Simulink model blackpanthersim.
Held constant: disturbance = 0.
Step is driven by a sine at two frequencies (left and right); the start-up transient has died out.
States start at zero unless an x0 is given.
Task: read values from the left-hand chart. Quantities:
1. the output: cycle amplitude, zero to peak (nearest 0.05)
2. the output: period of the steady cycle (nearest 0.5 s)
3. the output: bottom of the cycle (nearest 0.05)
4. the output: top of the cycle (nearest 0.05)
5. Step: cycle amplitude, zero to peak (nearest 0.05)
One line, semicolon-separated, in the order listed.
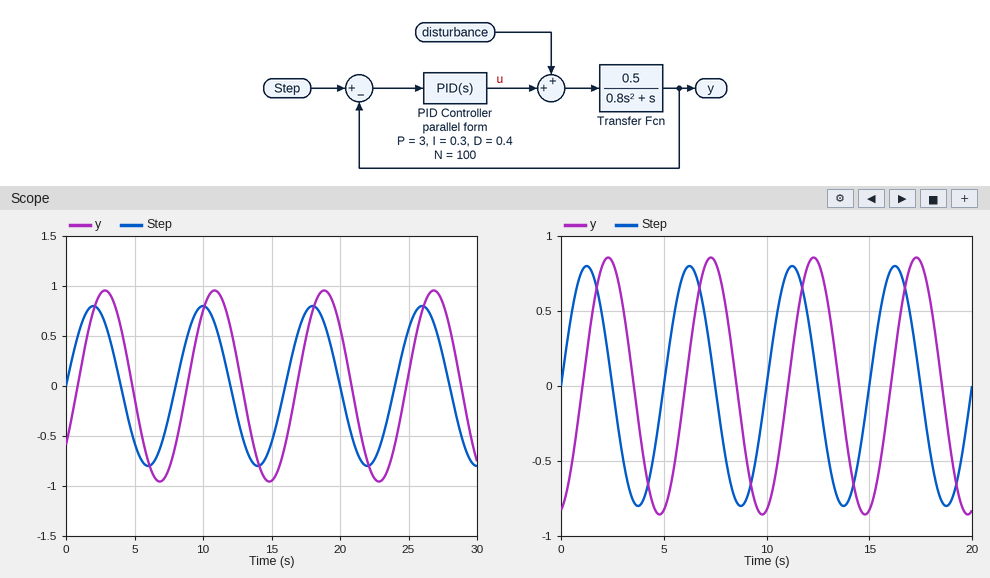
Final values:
0.95; 8.0 s; -0.95; 0.95; 0.80
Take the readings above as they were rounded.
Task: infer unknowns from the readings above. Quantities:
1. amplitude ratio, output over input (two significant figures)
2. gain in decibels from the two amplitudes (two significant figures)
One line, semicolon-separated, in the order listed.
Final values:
1.2; 1.5 dB
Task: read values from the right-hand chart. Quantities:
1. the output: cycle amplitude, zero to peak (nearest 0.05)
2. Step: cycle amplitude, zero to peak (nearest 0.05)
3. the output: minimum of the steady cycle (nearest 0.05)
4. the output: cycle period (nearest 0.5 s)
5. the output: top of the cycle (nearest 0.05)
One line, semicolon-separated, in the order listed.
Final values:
0.85; 0.80; -0.85; 5.0 s; 0.85
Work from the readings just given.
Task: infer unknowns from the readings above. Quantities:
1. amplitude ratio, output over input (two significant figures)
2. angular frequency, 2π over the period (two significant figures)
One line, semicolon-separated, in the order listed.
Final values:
1.1; 1.3 rad/s
